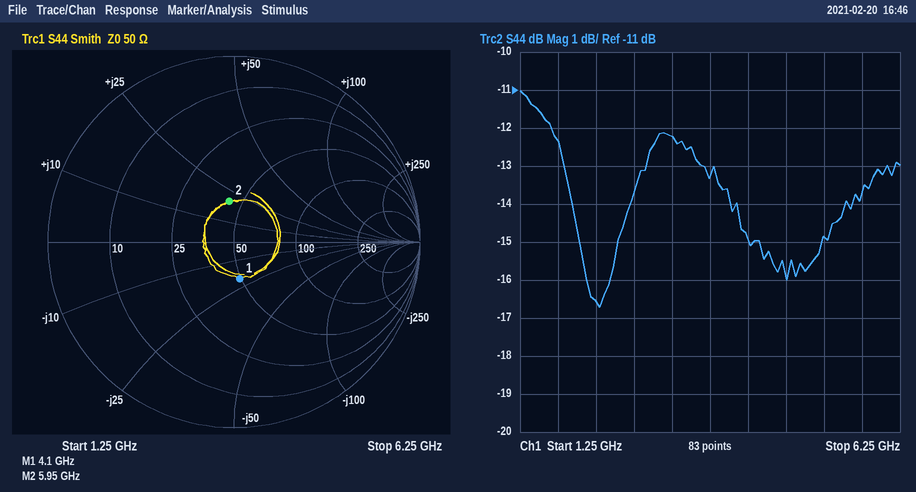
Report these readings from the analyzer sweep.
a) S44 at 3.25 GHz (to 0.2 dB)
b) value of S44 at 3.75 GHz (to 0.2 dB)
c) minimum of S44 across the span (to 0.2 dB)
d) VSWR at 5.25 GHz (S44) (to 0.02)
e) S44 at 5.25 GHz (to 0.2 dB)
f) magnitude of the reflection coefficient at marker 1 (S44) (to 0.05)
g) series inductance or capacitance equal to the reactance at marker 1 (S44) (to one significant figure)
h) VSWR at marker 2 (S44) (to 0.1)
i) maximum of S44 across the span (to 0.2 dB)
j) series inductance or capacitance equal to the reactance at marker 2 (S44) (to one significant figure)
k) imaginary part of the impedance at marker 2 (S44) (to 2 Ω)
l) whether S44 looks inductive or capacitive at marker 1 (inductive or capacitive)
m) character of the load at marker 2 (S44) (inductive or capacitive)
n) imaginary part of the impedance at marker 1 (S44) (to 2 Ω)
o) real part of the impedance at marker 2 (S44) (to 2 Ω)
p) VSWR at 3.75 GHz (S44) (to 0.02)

-12.2 dB
-13.2 dB
-16.8 dB
1.44
-14.8 dB
0.20
2 pF
1.6
-11.0 dB
500 pH
+20 Ω
capacitive
inductive
-20 Ω
44 Ω
1.56
